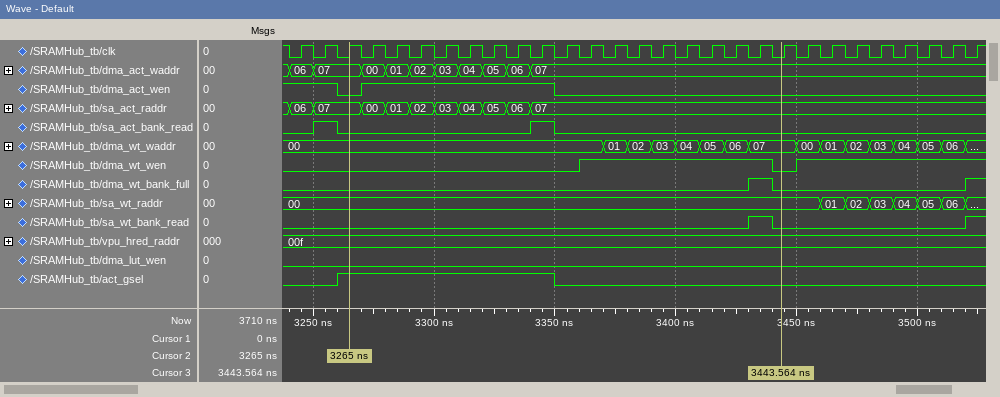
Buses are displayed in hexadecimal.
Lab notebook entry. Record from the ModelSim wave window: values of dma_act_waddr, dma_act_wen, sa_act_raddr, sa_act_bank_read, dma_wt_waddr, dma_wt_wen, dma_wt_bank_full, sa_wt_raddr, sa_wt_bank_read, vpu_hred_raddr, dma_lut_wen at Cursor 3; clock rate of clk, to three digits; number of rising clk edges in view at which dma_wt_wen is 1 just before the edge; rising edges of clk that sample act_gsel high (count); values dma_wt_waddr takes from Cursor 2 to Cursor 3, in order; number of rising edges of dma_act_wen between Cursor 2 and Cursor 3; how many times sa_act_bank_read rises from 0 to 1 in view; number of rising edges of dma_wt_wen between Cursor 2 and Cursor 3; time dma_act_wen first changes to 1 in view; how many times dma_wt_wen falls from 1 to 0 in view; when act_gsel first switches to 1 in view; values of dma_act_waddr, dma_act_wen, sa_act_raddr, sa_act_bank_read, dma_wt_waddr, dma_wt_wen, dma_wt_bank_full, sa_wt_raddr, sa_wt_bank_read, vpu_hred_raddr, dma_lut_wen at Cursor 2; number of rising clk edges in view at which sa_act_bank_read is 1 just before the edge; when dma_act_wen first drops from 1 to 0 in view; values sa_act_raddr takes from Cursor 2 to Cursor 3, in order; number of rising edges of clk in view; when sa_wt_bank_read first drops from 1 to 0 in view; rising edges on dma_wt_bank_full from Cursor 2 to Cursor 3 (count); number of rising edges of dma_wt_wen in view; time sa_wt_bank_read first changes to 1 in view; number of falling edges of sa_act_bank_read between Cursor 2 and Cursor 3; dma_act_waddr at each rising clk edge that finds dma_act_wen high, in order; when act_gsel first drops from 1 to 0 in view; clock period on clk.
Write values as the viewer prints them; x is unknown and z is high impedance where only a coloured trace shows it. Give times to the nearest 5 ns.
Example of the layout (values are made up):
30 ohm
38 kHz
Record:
dma_act_waddr=07, dma_act_wen=0, sa_act_raddr=07, sa_act_bank_read=0, dma_wt_waddr=07, dma_wt_wen=0, dma_wt_bank_full=0, sa_wt_raddr=00, sa_wt_bank_read=0, vpu_hred_raddr=00f, dma_lut_wen=0
100 MHz
16
9
00, 01, 02, 03, 04, 05, 06, 07
1
2
1
3270 ns
1
3260 ns
dma_act_waddr=07, dma_act_wen=0, sa_act_raddr=07, sa_act_bank_read=0, dma_wt_waddr=00, dma_wt_wen=0, dma_wt_bank_full=0, sa_wt_raddr=00, sa_wt_bank_read=0, vpu_hred_raddr=00f, dma_lut_wen=0
2
3260 ns
07, 00, 01, 02, 03, 04, 05, 06, 07
29
3440 ns
1
2
3430 ns
1
06, 07, 00, 01, 02, 03, 04, 05, 06, 07
3350 ns
10 ns
